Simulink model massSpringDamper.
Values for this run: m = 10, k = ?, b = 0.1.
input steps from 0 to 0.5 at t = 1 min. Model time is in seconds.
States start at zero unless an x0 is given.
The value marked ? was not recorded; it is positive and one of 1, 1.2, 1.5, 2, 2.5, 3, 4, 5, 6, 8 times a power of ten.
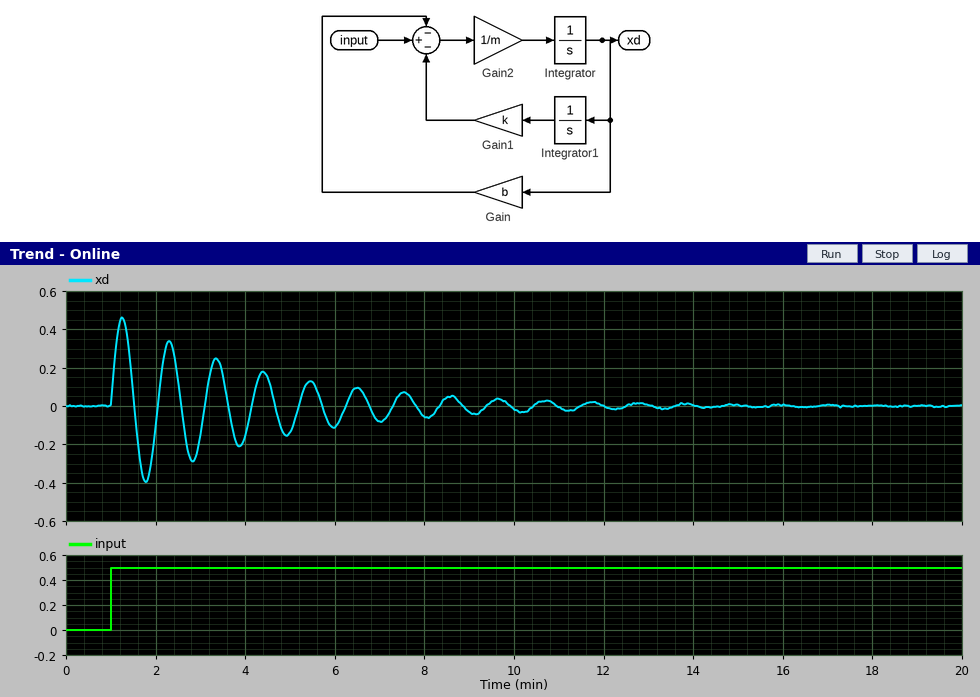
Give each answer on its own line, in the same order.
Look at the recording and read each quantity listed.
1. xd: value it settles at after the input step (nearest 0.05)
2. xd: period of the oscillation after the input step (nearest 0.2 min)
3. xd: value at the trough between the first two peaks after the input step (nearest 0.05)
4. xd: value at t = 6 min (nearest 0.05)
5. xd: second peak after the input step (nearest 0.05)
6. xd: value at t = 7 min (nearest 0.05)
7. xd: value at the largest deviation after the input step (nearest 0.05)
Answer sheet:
0.00
1.0 min
-0.40
-0.10
0.35
-0.10
0.45
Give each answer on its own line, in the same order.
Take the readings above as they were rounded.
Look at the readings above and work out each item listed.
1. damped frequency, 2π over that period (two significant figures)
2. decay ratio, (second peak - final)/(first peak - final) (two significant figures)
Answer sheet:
6.3 rad/min
0.78
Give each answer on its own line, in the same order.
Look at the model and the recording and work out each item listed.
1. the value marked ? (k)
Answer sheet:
0.1
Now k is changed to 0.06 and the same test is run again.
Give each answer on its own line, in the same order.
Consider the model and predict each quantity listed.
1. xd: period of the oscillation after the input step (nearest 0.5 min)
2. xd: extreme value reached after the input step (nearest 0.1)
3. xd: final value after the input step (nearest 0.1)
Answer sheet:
1.5 min
0.6
0.0
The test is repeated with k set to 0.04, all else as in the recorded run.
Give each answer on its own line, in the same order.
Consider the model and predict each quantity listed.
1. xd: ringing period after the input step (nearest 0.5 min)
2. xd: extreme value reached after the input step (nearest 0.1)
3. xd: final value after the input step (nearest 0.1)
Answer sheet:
1.5 min
0.7
0.0
